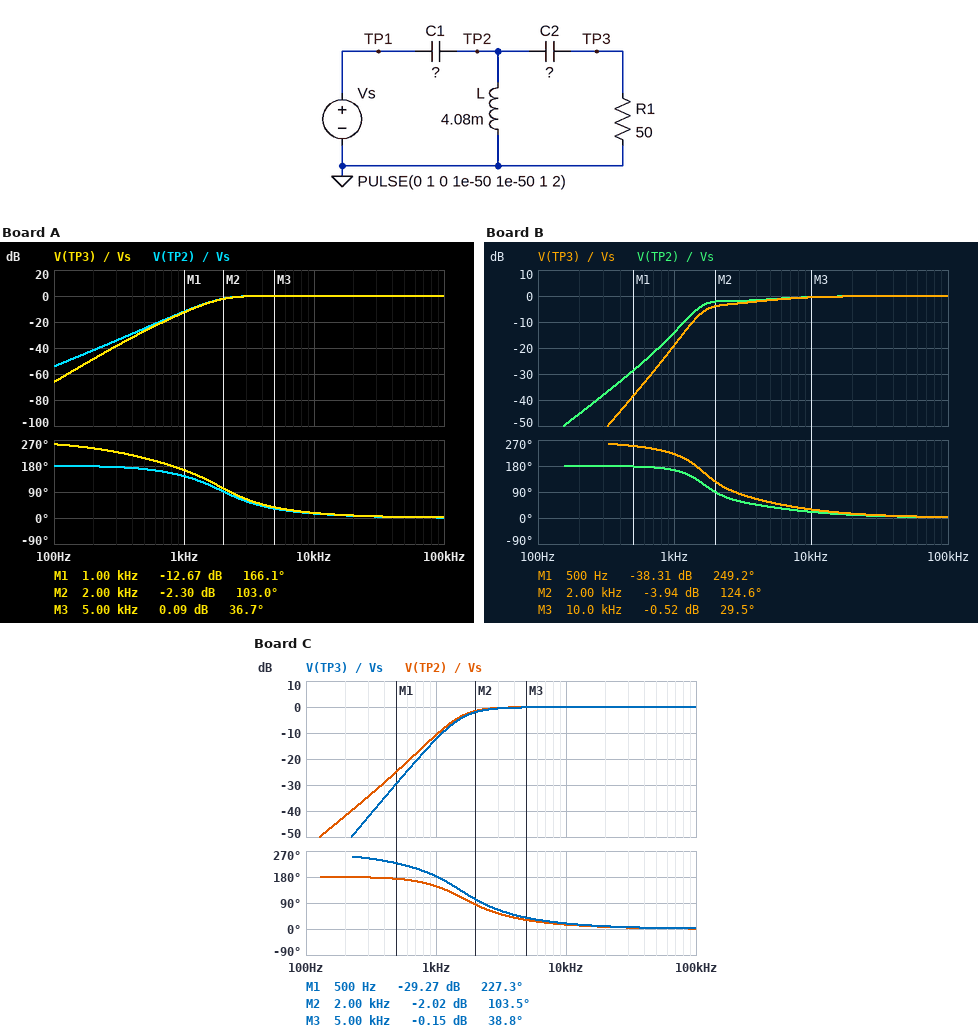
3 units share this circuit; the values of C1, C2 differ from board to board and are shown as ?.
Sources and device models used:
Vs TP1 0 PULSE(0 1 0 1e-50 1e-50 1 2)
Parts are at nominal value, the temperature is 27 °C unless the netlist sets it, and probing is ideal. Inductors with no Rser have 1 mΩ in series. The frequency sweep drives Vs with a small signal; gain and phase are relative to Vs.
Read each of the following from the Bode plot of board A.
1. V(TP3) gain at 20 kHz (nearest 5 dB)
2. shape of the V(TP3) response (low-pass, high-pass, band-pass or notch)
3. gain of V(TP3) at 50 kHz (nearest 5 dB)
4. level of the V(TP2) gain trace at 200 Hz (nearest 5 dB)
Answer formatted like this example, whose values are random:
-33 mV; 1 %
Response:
0 dB; high-pass; 0 dB; -40 dB
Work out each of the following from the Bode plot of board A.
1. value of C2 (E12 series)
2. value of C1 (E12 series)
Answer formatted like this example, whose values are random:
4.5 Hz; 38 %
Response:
8.2 µF; 1.2 µF
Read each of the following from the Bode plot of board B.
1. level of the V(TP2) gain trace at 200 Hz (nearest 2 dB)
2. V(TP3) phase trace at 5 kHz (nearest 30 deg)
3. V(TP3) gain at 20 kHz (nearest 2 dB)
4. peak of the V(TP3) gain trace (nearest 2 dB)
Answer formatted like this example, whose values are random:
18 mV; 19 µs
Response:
-46 dB; 60 deg; 0 dB; 0 dB
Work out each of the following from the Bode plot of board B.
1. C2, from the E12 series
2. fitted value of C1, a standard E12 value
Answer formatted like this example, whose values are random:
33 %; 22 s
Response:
2.2 µF; 820 nF
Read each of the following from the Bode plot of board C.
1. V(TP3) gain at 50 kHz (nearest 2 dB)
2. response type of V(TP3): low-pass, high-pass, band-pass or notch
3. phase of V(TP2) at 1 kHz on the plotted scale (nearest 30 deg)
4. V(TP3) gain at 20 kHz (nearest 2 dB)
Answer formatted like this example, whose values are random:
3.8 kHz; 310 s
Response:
0 dB; high-pass; 150 deg; 0 dB
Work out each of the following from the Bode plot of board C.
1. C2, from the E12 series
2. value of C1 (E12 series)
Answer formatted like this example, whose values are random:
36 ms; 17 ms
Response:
4.7 µF; 1.2 µF
